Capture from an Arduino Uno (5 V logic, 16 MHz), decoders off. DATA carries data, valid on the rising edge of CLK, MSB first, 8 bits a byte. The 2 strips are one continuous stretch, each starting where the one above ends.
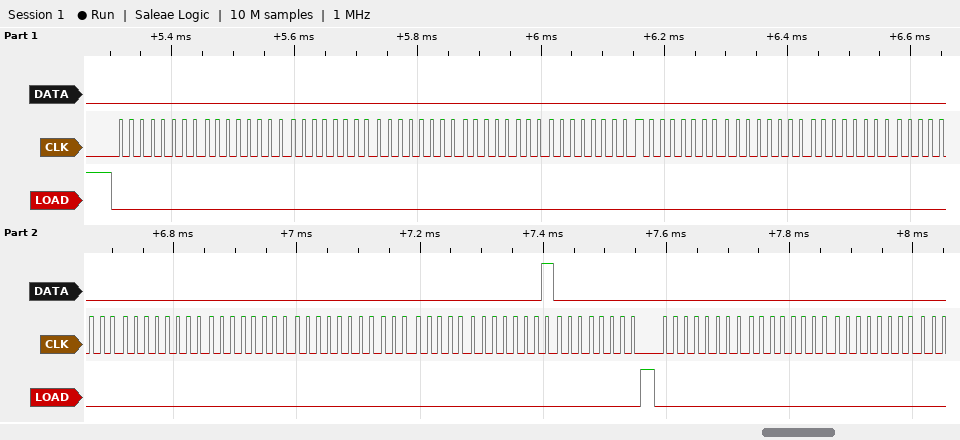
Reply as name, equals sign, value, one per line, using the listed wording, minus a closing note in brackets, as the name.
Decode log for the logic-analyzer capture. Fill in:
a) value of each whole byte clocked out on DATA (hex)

value of each whole byte clocked out on DATA = 00 00 00 00 00 00 00 00 00 00 00 00 00 00 01 00 00 00 00
